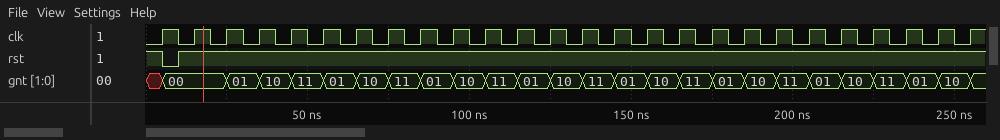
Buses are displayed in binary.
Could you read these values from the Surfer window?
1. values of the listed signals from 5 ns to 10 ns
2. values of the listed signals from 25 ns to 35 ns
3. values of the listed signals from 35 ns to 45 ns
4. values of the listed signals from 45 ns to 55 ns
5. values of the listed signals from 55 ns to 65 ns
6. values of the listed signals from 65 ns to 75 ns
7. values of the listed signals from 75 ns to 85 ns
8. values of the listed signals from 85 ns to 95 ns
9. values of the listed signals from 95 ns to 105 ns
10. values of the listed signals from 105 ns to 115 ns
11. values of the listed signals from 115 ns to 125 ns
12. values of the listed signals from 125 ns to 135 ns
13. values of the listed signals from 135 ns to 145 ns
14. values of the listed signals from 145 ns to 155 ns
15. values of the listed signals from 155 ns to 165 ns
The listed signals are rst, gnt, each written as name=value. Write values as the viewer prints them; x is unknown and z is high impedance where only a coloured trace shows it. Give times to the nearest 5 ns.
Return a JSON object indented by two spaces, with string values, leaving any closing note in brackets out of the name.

{
  "values of the listed signals from 5 ns to 10 ns": "rst=0, gnt=00",
  "values of the listed signals from 25 ns to 35 ns": "rst=1, gnt=01",
  "values of the listed signals from 35 ns to 45 ns": "rst=1, gnt=10",
  "values of the listed signals from 45 ns to 55 ns": "rst=1, gnt=11",
  "values of the listed signals from 55 ns to 65 ns": "rst=1, gnt=01",
  "values of the listed signals from 65 ns to 75 ns": "rst=1, gnt=10",
  "values of the listed signals from 75 ns to 85 ns": "rst=1, gnt=11",
  "values of the listed signals from 85 ns to 95 ns": "rst=1, gnt=01",
  "values of the listed signals from 95 ns to 105 ns": "rst=1, gnt=10",
  "values of the listed signals from 105 ns to 115 ns": "rst=1, gnt=11",
  "values of the listed signals from 115 ns to 125 ns": "rst=1, gnt=01",
  "values of the listed signals from 125 ns to 135 ns": "rst=1, gnt=10",
  "values of the listed signals from 135 ns to 145 ns": "rst=1, gnt=11",
  "values of the listed signals from 145 ns to 155 ns": "rst=1, gnt=01",
  "values of the listed signals from 155 ns to 165 ns": "rst=1, gnt=10"
}
